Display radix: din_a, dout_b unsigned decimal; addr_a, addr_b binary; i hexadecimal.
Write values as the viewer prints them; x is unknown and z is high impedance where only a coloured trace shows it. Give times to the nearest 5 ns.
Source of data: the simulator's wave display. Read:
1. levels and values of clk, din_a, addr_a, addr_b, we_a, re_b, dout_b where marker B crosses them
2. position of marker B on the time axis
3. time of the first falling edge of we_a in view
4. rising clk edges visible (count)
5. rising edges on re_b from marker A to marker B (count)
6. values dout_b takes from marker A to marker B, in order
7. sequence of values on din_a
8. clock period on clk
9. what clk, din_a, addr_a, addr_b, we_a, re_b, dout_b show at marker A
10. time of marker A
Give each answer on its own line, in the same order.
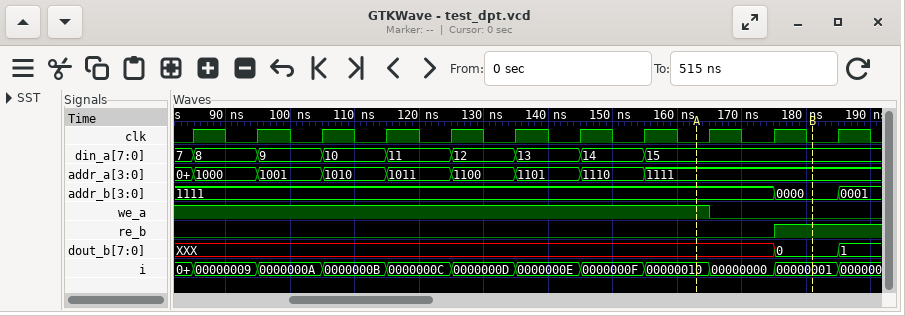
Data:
clk=0, din_a=15, addr_a=1111, addr_b=0000, we_a=0, re_b=1, dout_b=0
180 ns
165 ns
11
1
XXX, 0
7, 8, 9, 10, 11, 12, 13, 14, 15
10 ns
clk=0, din_a=15, addr_a=1111, addr_b=1111, we_a=1, re_b=0, dout_b=XXX
165 ns
